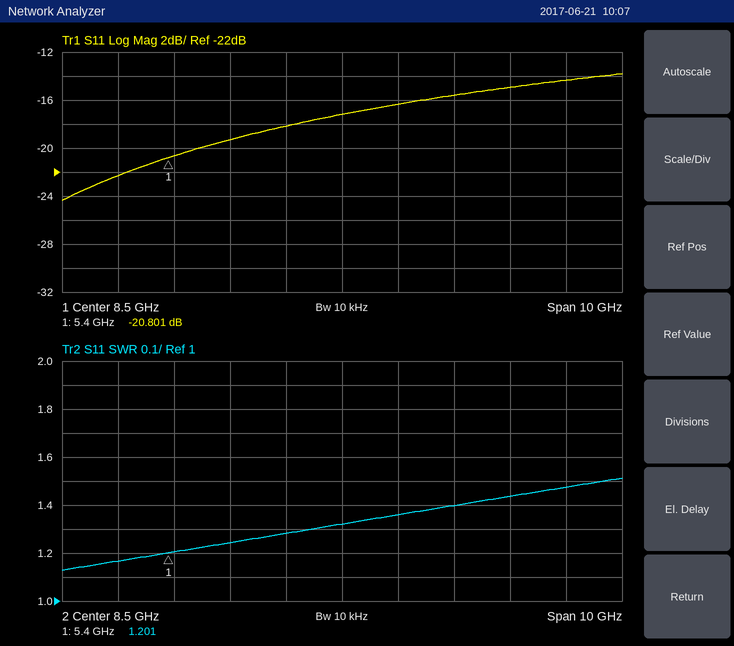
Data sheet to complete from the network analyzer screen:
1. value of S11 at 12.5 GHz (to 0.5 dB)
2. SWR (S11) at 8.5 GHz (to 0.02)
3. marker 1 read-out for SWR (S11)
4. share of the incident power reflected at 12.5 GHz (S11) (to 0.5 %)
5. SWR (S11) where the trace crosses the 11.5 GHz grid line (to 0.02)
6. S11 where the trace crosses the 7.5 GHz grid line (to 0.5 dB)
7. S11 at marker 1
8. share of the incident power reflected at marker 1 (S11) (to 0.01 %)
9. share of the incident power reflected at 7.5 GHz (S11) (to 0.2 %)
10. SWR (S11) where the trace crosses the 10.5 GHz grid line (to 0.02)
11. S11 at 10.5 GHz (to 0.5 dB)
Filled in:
-14.5 dB
1.32
1.201
3.5 %
1.44
-18.0 dB
-20.801 dB
0.83 %
1.6 %
1.40
-15.5 dB
